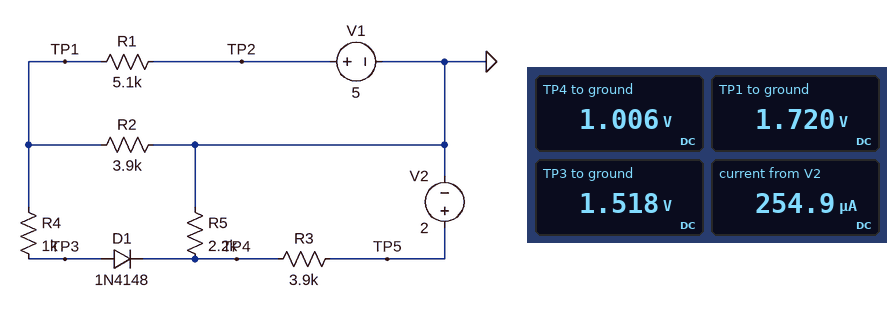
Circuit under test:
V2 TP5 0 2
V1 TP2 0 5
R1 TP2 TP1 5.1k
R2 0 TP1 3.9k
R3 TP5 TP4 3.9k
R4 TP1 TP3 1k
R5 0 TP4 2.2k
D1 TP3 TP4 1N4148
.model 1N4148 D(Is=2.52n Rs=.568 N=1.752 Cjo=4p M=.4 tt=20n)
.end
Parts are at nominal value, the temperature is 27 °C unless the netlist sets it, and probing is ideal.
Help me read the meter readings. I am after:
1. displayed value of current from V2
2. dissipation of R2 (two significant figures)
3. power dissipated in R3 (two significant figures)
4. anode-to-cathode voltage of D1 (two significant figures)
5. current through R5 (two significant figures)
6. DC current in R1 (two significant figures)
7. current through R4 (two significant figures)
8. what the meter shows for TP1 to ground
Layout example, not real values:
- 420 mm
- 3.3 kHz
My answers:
- 254.9 µA
- 760 µW
- 250 µW
- 510 mV
- 460 µA
- 640 µA
- 200 µA
- 1.720 V
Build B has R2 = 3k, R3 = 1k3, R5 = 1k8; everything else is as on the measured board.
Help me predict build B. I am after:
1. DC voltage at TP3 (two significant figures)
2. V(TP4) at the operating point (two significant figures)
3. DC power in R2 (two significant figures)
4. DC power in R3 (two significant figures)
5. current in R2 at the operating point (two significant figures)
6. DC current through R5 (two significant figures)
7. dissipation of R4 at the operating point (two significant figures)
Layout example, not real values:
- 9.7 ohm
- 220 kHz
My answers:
- 1.7 V
- 1.2 V
- 1.0 mW
- 480 µW
- 580 µA
- 670 µA
- 4.0 µW
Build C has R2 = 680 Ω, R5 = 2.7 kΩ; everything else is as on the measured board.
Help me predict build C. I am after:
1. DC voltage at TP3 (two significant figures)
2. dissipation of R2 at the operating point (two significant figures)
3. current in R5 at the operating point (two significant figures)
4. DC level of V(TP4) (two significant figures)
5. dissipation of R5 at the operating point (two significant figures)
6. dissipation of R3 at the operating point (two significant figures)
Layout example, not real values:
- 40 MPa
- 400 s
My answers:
- 590 mV
- 510 µW
- 300 µA
- 820 mV
- 250 µW
- 360 µW
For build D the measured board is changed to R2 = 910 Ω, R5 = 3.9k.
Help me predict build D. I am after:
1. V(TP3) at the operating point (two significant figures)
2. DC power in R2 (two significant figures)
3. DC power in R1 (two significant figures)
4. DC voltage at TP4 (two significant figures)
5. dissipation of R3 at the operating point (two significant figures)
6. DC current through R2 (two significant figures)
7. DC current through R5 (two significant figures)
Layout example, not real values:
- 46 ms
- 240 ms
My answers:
- 760 mV
- 630 µW
- 3.5 mW
- 1.0 V
- 260 µW
- 830 µA
- 260 µA
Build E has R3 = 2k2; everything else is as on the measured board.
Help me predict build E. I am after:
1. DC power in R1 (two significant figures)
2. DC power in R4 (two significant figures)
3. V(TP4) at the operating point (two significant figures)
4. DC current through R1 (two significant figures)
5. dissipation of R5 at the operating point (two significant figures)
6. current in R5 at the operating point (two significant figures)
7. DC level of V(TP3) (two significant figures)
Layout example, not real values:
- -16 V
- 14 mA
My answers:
- 2.0 mW
- 24 µW
- 1.2 V
- 620 µA
- 620 µW
- 530 µA
- 1.7 V
